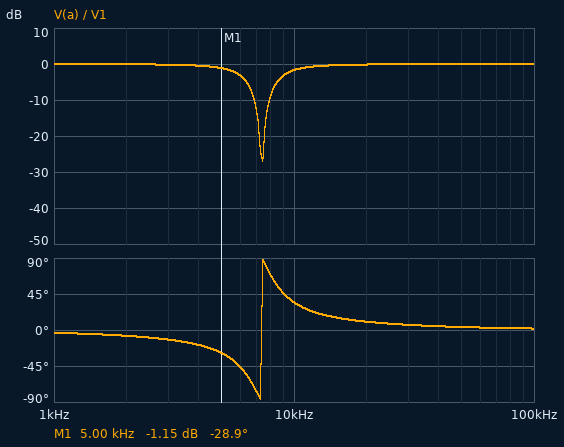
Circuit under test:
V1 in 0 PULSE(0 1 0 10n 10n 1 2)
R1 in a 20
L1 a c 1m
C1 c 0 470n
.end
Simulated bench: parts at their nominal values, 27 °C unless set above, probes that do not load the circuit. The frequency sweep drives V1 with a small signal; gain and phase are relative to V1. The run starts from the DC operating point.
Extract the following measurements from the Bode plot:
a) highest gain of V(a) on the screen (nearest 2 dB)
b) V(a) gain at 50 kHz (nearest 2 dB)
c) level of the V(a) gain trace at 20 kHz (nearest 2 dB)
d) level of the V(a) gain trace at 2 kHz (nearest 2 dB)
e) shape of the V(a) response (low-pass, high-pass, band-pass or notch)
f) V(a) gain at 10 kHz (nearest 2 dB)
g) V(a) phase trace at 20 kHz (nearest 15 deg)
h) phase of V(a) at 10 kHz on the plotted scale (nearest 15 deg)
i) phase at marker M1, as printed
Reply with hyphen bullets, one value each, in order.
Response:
- 0 dB
- 0 dB
- 0 dB
- 0 dB
- notch
- -2 dB
- 15 deg
- 30 deg
- -28.9 deg
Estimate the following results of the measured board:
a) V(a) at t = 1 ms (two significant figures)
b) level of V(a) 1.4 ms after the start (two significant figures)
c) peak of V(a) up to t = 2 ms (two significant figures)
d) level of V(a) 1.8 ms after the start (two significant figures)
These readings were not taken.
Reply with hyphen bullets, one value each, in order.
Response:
- 1.0 V
- 1.0 V
- 1.2 V
- 1.0 V
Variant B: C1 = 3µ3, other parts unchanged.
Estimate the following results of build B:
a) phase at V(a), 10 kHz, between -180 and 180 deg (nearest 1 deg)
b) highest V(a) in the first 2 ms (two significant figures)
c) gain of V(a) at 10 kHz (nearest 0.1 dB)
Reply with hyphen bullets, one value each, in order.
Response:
- 19 deg
- 1.1 V
- -0.5 dB
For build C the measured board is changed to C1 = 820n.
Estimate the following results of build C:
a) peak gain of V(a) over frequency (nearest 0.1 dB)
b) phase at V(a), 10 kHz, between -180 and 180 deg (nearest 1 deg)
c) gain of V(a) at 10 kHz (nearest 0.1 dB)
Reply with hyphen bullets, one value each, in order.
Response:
- 0 dB
- 25 deg
- -0.8 dB
